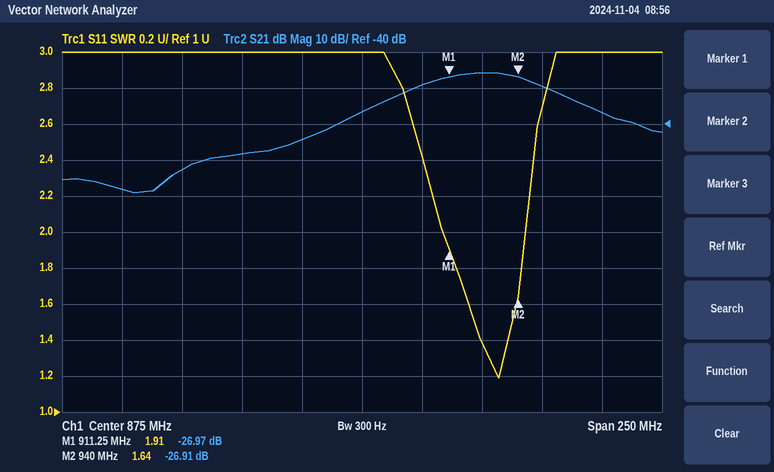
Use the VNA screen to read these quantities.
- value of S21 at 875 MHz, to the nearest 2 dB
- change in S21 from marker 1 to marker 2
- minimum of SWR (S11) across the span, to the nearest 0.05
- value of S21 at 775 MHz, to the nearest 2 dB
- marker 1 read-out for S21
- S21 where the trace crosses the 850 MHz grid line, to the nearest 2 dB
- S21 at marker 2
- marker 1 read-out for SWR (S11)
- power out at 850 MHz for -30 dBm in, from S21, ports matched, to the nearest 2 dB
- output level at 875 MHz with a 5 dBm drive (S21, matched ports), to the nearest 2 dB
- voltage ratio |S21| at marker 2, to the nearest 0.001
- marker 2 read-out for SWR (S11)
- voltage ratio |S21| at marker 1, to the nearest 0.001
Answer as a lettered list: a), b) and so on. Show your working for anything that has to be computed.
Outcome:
a) -36 dB
b) -26.91 − (-26.97) = 0.06 dB
c) 1.20
d) -58 dB
e) -26.97 dB
f) -44 dB
g) -26.91 dB
h) 1.91
i) -30 dBm + (-44 dB) = -74 dBm
j) 5 dBm + (-36 dB) = -32 dBm
k) 10^(-26.91/20) ≈ 0.045
l) 1.64
m) 10^(-26.97/20) ≈ 0.045
